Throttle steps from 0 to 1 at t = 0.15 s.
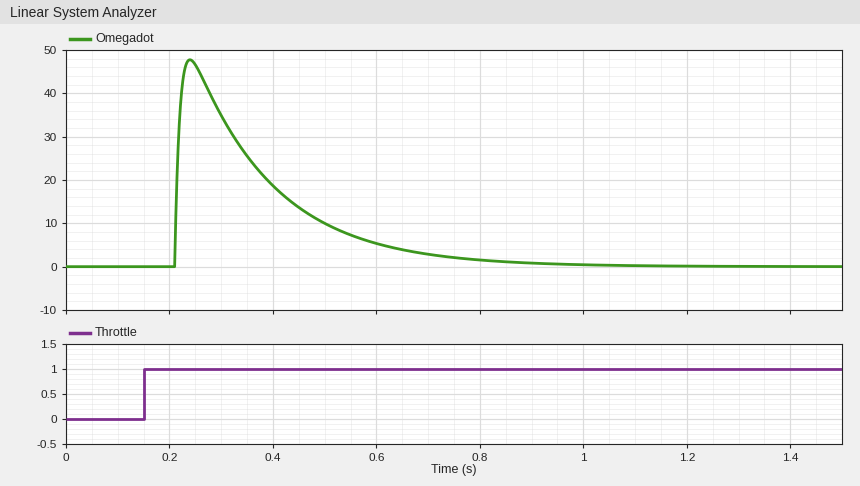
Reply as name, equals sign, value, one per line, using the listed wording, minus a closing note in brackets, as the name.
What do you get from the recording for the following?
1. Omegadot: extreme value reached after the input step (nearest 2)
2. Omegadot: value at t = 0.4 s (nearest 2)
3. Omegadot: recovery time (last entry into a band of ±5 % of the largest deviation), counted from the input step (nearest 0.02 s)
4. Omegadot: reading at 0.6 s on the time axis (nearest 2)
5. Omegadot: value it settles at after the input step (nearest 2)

Omegadot: extreme value reached after the input step = 48
Omegadot: value at t = 0.4 s = 18
Omegadot: recovery time (last entry into a band of ±5 % of the largest deviation), counted from the input step = 0.58 s
Omegadot: reading at 0.6 s on the time axis = 6
Omegadot: value it settles at after the input step = 0
